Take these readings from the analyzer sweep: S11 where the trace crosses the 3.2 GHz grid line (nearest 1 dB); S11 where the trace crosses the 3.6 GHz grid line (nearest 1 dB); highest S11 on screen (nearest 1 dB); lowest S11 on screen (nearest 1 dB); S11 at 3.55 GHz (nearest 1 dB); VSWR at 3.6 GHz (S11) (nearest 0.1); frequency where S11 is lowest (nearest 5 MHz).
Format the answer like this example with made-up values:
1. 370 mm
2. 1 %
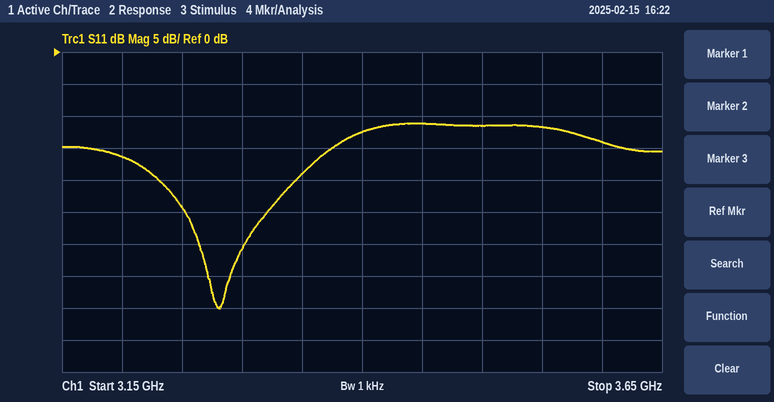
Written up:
1. -16 dB
2. -14 dB
3. -11 dB
4. -40 dB
5. -12 dB
6. 1.5
7. 3.280 GHz
